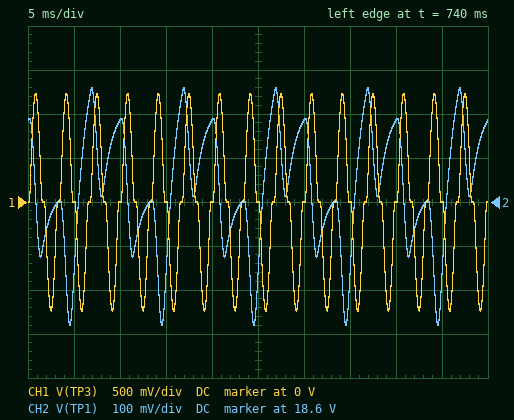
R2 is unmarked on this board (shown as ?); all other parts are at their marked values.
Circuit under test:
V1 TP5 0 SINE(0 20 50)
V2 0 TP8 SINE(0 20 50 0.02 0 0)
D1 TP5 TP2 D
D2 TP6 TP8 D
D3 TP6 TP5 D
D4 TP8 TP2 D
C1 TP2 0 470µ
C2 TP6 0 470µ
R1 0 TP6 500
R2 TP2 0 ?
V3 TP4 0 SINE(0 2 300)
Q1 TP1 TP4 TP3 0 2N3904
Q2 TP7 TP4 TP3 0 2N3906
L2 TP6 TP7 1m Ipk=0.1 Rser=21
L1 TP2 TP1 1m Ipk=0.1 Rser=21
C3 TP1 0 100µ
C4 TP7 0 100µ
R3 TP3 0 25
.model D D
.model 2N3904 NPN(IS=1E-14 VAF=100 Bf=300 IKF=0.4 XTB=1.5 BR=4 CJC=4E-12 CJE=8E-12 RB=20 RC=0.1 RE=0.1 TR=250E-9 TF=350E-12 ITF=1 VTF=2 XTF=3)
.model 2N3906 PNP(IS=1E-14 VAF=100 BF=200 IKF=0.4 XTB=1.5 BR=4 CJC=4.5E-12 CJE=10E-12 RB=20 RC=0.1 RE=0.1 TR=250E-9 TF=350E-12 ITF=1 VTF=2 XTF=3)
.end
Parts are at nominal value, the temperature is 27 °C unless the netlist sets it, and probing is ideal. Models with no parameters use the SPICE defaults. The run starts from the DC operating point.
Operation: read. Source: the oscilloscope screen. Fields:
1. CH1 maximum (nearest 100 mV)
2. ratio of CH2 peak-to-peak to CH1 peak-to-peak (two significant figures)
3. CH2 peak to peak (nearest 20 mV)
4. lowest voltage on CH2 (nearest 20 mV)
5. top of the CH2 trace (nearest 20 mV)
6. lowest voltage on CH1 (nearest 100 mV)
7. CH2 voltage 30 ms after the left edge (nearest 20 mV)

1.2 V
0.22
540 mV
18.32 V
18.86 V
-1.2 V
18.78 V
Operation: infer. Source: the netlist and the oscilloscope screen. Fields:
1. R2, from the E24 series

820 Ω
